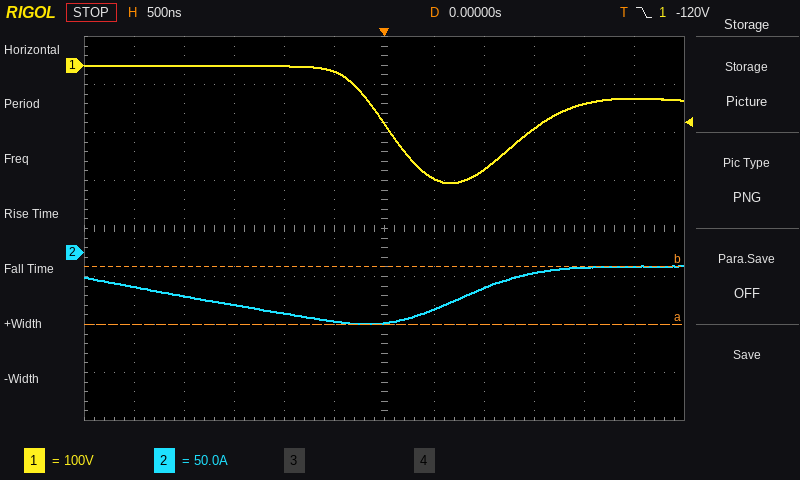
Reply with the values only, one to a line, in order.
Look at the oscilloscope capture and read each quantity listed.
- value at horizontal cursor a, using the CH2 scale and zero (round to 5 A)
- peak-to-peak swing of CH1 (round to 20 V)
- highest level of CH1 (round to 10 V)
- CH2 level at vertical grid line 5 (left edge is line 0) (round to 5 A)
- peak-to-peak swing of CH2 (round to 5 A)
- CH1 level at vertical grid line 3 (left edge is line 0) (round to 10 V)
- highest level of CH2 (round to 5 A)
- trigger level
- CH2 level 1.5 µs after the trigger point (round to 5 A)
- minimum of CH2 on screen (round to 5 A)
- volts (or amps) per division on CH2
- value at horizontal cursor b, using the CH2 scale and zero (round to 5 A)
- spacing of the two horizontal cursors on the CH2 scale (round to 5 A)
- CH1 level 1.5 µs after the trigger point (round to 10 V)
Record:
-75 A
240 V
0 V
-70 A
60 A
0 V
-15 A
-120 V
-20 A
-75 A
50 A
-15 A
60 A
-130 V
